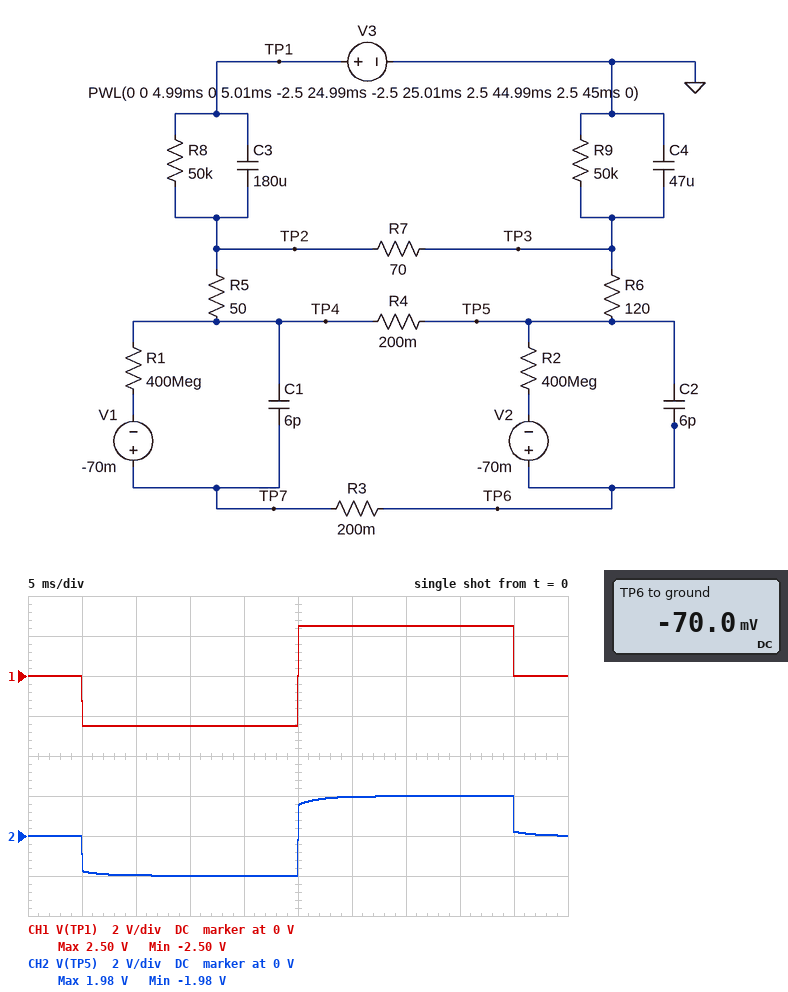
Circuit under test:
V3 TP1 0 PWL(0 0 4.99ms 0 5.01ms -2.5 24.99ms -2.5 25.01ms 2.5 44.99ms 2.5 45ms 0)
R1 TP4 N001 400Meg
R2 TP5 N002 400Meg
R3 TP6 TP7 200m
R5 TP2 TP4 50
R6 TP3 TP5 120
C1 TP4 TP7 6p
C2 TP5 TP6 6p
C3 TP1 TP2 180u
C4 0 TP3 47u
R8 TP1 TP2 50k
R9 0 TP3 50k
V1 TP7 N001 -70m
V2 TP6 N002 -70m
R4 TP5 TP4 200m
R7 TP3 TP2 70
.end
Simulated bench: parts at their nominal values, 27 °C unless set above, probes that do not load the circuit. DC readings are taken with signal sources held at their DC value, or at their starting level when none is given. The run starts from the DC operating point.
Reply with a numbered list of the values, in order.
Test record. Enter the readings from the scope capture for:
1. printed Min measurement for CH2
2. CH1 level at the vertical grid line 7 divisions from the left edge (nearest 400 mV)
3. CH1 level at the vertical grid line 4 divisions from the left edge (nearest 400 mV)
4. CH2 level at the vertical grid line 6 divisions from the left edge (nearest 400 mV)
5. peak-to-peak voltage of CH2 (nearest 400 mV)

1. -1.98 V
2. 2.4 V
3. -2.4 V
4. 2.0 V
5. 4.0 V
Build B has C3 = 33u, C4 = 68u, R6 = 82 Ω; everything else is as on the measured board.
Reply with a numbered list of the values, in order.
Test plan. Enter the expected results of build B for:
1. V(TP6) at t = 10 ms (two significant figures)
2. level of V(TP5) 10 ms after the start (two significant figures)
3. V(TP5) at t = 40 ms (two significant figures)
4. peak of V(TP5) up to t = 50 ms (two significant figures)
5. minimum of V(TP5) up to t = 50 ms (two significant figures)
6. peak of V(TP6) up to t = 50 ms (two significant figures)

1. -890 mV
2. -820 mV
3. 820 mV
4. 2.3 V
5. -1.5 V
6. 2.2 V
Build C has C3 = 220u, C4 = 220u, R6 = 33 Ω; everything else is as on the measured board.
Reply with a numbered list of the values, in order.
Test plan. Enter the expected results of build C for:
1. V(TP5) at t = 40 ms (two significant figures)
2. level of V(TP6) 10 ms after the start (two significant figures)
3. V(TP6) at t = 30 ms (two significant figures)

1. 1.2 V
2. -1.2 V
3. 1.0 V
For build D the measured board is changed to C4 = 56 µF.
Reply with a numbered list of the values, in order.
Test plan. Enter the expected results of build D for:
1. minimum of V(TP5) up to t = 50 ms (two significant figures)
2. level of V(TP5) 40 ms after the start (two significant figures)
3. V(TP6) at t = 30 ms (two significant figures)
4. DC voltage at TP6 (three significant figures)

1. -1.9 V
2. 1.9 V
3. 1.8 V
4. -70.0 mV
